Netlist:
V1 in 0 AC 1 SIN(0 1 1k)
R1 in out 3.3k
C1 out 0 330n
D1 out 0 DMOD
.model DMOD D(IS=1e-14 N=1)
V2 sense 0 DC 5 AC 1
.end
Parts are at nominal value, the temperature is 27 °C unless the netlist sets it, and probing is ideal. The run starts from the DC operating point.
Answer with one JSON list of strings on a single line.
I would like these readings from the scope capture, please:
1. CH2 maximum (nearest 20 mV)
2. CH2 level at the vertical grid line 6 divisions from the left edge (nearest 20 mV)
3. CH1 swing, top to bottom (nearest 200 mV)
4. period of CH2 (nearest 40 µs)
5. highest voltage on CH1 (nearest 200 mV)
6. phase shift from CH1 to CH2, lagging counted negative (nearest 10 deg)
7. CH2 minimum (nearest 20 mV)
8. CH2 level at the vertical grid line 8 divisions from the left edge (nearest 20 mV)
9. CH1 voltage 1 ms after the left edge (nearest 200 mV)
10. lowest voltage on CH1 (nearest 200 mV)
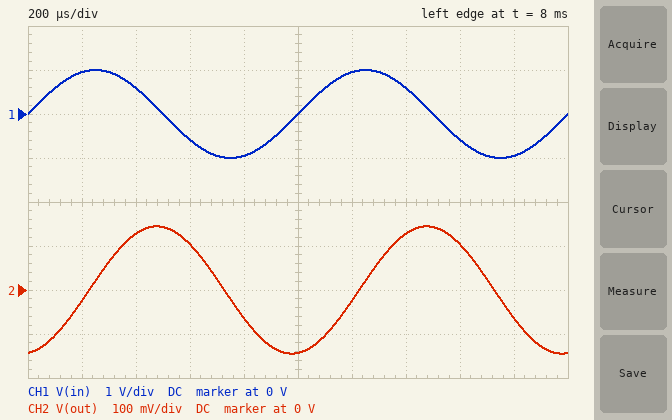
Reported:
["140 mV", "-20 mV", "2.0 V", "1.00 ms", "1.0 V", "-80 deg", "-140 mV", "100 mV", "0 V", "-1.0 V"]
